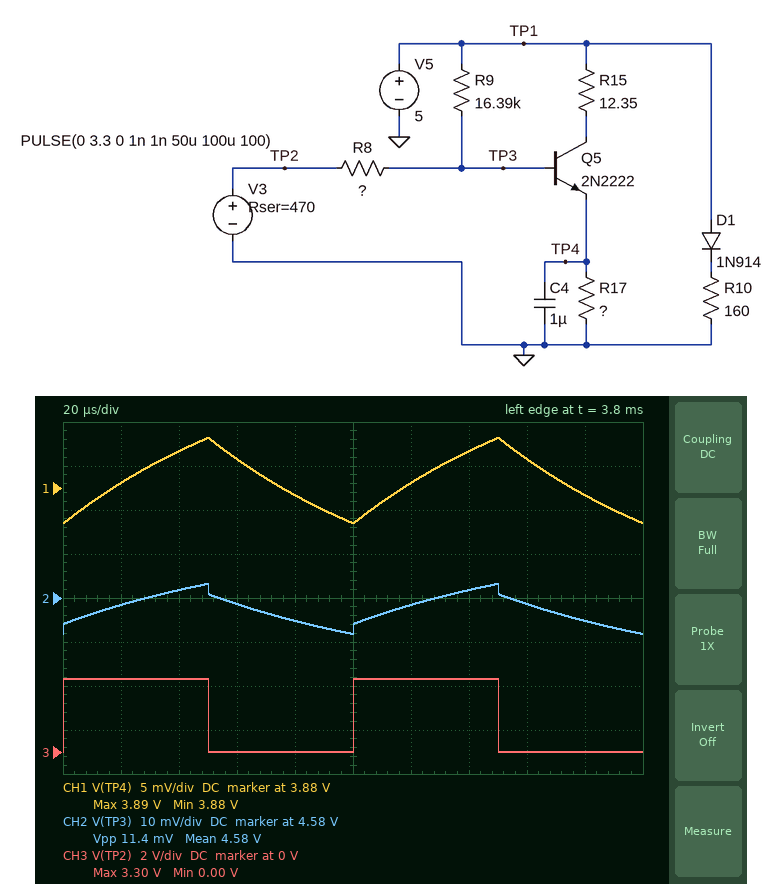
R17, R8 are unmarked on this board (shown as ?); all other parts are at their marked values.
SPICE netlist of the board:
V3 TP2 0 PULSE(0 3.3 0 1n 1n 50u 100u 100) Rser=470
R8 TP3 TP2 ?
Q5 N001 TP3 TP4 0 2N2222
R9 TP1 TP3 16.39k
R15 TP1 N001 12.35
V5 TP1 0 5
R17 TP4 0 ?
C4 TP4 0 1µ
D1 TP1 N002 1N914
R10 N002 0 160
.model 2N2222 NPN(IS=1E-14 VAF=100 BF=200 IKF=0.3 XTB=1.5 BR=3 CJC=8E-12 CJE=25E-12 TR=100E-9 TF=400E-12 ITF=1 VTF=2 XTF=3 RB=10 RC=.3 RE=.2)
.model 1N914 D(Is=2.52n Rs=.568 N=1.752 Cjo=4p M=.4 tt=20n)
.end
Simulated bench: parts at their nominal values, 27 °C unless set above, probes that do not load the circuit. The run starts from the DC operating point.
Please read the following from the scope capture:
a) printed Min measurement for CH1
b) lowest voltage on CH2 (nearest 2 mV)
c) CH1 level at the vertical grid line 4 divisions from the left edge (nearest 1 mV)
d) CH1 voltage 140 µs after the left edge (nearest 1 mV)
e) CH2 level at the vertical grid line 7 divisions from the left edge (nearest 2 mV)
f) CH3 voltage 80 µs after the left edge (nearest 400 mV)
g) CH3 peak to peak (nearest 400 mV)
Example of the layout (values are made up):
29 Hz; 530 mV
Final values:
3.88 V; 4.572 V; 3.879 V; 3.884 V; 4.582 V; 0 V; 3.2 V
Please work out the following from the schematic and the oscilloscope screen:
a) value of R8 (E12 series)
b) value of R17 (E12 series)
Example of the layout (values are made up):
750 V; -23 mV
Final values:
1.5 MΩ; 820 Ω
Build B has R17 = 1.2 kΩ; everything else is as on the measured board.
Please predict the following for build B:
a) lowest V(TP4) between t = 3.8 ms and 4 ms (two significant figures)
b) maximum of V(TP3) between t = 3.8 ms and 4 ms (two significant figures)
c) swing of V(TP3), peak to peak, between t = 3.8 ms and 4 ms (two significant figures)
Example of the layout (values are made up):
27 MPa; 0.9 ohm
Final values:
4.0 V; 4.7 V; 12 mV
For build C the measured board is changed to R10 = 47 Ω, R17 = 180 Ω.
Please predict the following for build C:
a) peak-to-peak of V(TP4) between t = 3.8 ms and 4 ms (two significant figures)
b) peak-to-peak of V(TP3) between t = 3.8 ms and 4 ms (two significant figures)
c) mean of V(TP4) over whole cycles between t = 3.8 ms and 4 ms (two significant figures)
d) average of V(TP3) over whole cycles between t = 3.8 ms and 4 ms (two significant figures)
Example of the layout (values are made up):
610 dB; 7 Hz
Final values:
9.3 mV; 9.9 mV; 2.9 V; 3.6 V
